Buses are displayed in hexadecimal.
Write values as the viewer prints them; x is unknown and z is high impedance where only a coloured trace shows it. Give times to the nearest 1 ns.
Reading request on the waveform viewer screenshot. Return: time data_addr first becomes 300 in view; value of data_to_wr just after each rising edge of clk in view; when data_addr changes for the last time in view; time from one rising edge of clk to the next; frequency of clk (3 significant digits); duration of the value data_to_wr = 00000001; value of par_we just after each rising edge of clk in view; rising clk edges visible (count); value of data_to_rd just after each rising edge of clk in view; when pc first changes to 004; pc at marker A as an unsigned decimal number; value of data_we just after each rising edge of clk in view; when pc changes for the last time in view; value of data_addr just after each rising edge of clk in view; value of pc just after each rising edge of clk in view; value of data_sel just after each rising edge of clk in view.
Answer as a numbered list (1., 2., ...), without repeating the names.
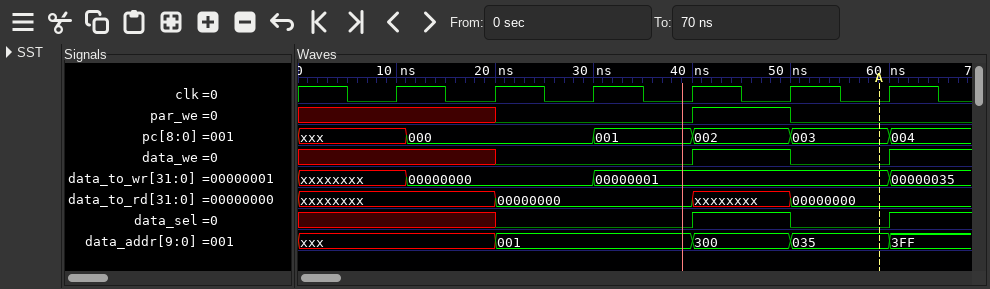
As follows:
1. 40 ns
2. xxxxxxxx, 00000000, 00000001, 00000001, 00000001, 00000035
3. 60 ns
4. 10 ns
5. 100 MHz
6. 30 ns
7. x 0 0 1 0 0
8. 6
9. xxxxxxxx, 00000000, 00000000, xxxxxxxx, 00000000, 00000000
10. 60 ns
11. 3
12. x 0 0 1 0 1
13. 60 ns
14. xxx, 001, 001, 300, 035, 3FF
15. xxx, 000, 001, 002, 003, 004
16. x 0 0 1 0 1
